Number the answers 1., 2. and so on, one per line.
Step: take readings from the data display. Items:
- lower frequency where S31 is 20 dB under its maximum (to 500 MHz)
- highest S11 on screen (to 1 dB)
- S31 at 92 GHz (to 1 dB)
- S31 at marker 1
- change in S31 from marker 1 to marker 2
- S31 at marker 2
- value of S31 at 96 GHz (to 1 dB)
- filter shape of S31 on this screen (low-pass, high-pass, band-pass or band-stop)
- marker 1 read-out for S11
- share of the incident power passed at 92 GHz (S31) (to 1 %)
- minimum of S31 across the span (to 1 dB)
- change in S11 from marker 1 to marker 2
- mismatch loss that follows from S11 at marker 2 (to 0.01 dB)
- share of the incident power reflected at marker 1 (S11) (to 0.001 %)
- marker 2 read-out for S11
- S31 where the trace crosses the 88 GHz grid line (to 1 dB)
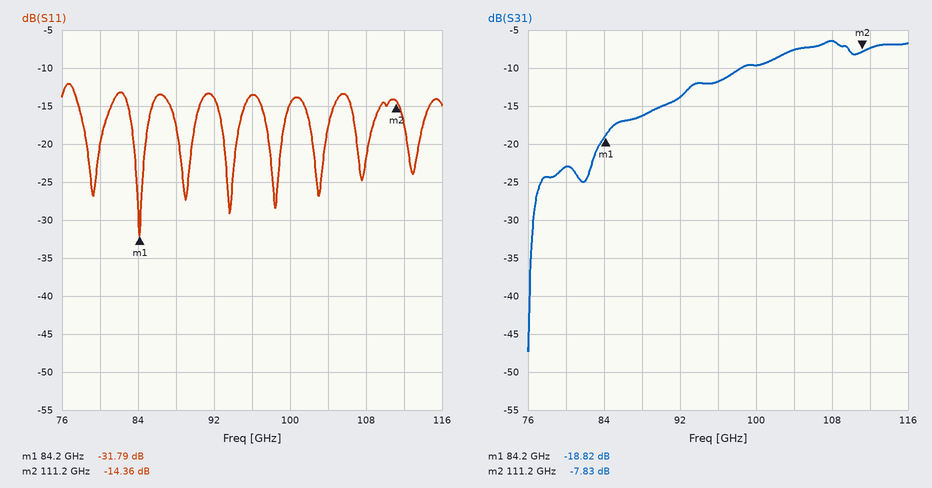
1. 77.0 GHz
2. -12 dB
3. -14 dB
4. -18.82 dB
5. 10.99 dB
6. -7.83 dB
7. -12 dB
8. high-pass
9. -31.79 dB
10. 4 %
11. -47 dB
12. 17.43 dB
13. 0.16 dB
14. 0.066 %
15. -14.36 dB
16. -16 dB
